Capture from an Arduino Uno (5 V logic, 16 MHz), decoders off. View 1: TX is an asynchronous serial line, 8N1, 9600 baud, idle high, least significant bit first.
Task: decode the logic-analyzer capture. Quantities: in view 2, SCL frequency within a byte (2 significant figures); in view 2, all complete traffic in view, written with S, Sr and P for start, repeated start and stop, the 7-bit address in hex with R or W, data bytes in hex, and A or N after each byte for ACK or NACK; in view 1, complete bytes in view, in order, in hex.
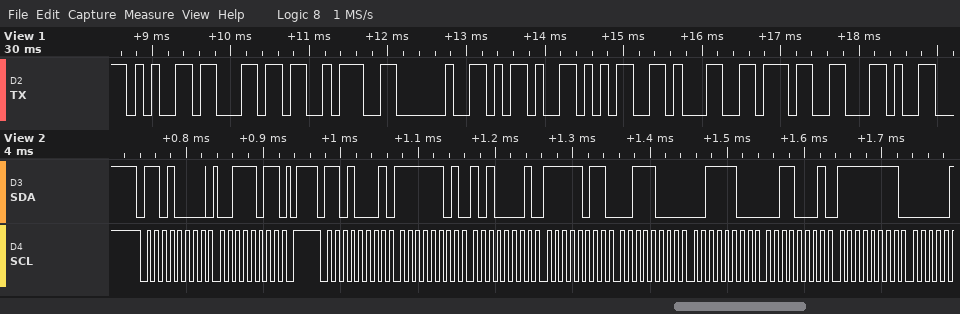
100 kHz
S 68W A 3B A P S 68R A FD A A1 A FB A 38 A 3C A 31 A FF A
0x65 0x6C 0x3A 0x20 0x2D 0x35 0x31 0x37 0x2C
